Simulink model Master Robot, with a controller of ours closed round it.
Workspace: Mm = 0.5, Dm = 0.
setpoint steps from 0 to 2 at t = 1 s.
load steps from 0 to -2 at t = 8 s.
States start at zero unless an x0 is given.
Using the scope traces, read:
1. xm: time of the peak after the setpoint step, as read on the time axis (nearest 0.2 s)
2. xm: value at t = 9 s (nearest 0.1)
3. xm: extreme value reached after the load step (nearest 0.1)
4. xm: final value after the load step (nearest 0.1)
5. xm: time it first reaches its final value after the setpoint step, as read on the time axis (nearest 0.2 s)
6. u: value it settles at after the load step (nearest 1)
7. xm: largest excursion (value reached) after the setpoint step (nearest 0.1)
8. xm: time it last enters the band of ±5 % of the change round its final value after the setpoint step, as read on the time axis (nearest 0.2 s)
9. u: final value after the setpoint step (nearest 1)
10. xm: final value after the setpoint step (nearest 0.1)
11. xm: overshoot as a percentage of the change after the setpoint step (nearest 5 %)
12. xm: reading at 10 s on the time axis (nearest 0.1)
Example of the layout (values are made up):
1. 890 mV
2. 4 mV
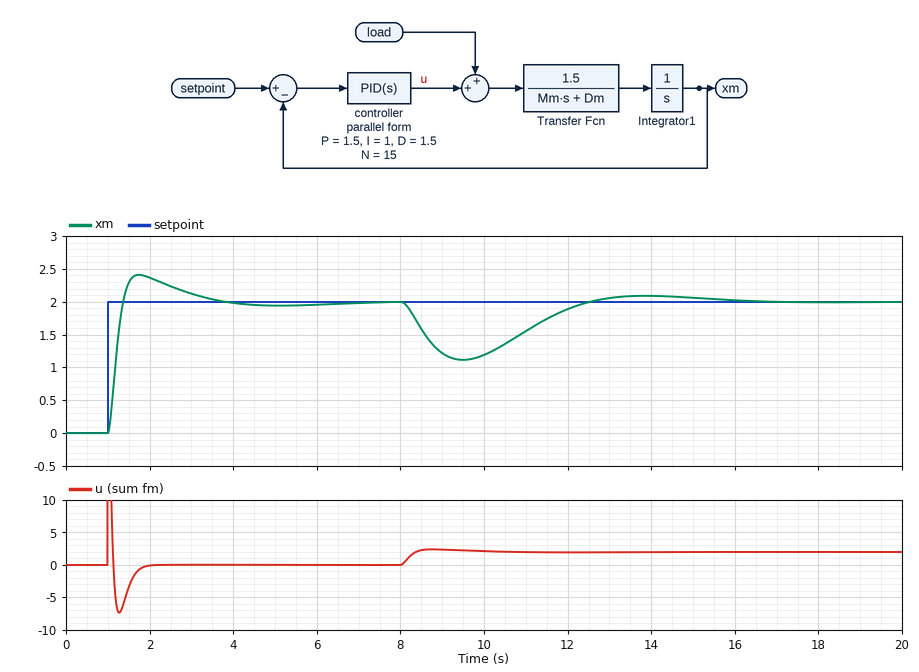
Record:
1. 1.8 s
2. 1.2
3. 1.1
4. 2.0
5. 1.4 s
6. 2
7. 2.4
8. 3.2 s
9. 0
10. 2.0
11. 20 %
12. 1.2
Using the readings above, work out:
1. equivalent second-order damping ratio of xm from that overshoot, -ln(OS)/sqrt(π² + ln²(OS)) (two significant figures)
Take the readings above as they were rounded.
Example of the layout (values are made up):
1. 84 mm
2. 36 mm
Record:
1. 0.46
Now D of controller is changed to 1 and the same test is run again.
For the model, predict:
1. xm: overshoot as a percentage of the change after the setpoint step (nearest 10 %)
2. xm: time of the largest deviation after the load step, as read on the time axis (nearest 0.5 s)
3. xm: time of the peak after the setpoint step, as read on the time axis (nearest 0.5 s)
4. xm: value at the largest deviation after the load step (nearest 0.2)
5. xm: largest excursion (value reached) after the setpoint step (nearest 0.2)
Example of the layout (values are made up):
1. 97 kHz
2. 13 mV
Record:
1. 30 %
2. 9.5 s
3. 2.0 s
4. 1.0
5. 2.6
